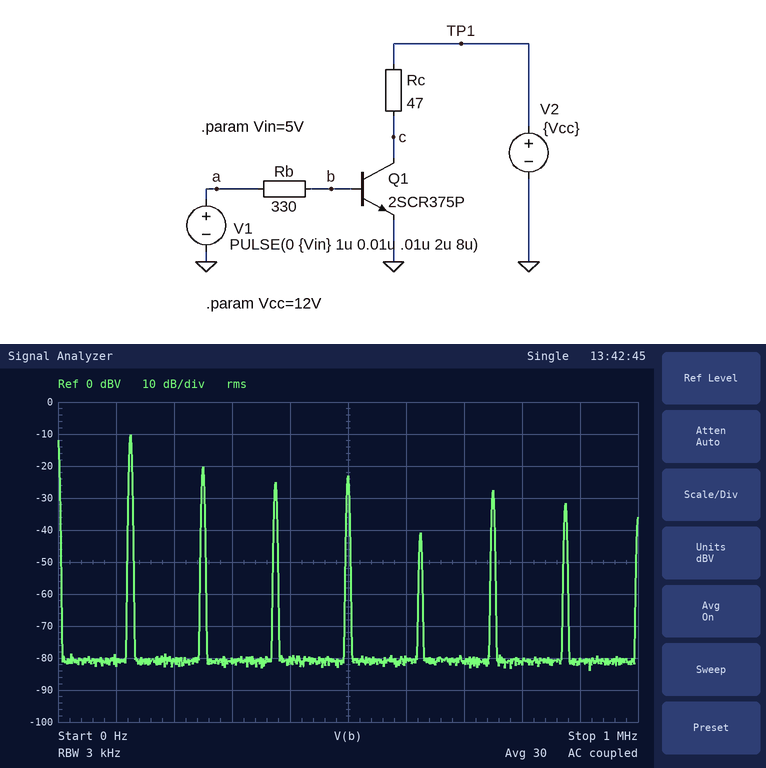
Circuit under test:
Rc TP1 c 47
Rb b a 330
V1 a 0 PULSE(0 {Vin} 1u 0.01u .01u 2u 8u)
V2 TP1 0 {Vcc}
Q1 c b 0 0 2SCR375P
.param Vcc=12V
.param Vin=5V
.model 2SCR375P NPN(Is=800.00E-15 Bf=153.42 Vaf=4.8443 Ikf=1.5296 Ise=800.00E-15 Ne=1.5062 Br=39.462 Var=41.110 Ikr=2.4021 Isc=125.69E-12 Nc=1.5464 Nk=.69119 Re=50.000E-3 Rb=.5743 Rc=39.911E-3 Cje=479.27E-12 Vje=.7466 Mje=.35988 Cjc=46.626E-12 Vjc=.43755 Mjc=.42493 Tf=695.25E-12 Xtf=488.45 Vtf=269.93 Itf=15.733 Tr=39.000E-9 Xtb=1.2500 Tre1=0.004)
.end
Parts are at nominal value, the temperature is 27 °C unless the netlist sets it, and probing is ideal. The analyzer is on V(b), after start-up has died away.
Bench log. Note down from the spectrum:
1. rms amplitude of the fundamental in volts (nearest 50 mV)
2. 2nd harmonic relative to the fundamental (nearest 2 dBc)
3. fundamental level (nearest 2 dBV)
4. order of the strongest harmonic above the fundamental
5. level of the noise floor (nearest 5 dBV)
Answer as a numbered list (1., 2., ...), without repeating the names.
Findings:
1. 300 mV
2. -10 dBc
3. -10 dBV
4. 2
5. -80 dBV
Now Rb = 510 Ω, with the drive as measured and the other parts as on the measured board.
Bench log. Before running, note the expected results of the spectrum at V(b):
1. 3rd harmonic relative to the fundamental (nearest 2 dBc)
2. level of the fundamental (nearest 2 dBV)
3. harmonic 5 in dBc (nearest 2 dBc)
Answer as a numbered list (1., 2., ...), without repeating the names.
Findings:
1. -16 dBc
2. -10 dBV
3. -24 dBc
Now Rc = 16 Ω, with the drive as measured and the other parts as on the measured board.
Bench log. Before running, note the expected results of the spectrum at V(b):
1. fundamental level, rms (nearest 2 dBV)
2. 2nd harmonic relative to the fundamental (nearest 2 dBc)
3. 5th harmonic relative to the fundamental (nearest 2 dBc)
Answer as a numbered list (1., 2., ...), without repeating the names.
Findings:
1. -10 dBV
2. -6 dBc
3. -16 dBc
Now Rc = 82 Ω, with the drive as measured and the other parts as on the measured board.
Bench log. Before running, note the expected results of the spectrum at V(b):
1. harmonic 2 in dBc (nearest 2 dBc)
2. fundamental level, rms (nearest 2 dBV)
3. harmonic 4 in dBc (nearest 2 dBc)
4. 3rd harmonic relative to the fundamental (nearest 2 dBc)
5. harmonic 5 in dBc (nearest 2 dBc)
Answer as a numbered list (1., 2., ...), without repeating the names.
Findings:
1. -12 dBc
2. -10 dBV
3. -14 dBc
4. -12 dBc
5. -22 dBc
